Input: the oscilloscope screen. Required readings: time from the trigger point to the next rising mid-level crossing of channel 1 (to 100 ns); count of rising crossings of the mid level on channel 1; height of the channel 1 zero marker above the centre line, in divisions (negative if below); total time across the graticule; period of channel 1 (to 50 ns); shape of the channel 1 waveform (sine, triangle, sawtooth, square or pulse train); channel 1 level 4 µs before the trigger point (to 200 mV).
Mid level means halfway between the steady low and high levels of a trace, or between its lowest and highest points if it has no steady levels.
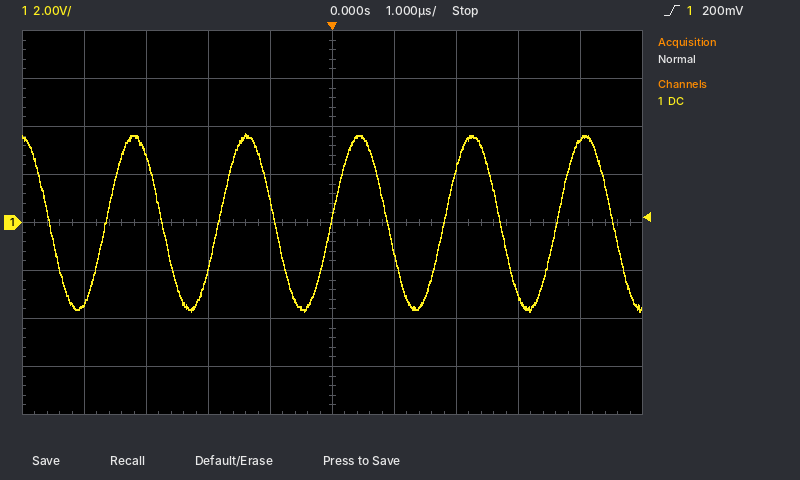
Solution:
1.8 µs
5
0.0 div
10 µs
1.80 µs
sine
-3.4 V
